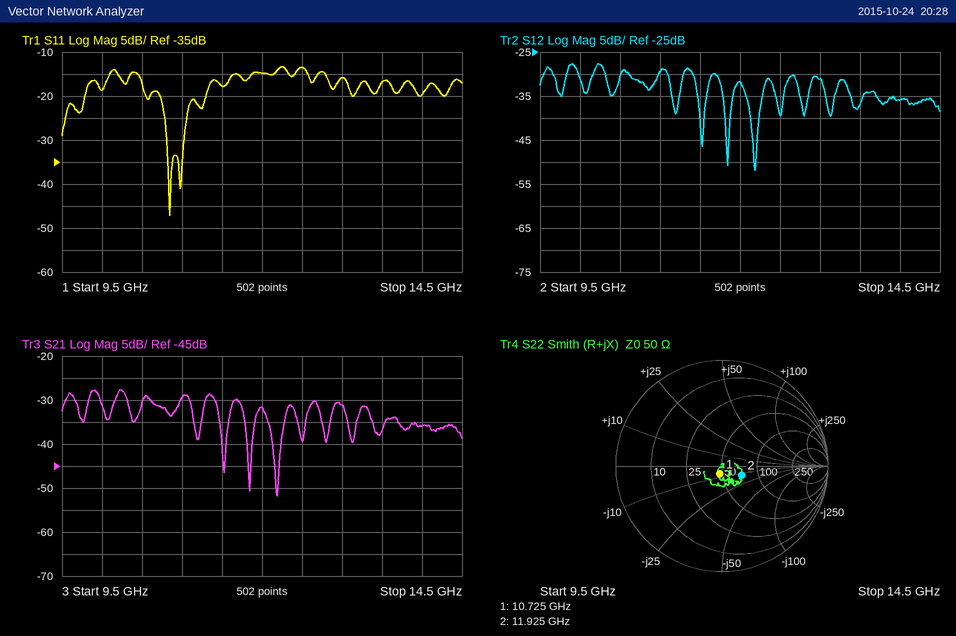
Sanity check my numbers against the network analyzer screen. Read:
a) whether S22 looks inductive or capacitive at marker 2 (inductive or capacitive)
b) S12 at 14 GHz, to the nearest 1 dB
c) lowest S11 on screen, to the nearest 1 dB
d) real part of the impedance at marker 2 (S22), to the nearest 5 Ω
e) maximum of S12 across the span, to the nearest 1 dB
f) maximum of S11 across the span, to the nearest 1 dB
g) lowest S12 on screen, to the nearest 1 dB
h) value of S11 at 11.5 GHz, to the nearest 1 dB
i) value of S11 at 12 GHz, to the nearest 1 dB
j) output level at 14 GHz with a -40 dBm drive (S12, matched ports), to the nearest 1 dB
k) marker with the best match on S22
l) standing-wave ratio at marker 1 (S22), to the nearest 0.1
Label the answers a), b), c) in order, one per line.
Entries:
a) capacitive
b) -36 dB
c) -47 dB
d) 70 Ω
e) -28 dB
f) -13 dB
g) -52 dB
h) -18 dB
i) -15 dB
j) -76 dBm
k) marker 1
l) 1.2
